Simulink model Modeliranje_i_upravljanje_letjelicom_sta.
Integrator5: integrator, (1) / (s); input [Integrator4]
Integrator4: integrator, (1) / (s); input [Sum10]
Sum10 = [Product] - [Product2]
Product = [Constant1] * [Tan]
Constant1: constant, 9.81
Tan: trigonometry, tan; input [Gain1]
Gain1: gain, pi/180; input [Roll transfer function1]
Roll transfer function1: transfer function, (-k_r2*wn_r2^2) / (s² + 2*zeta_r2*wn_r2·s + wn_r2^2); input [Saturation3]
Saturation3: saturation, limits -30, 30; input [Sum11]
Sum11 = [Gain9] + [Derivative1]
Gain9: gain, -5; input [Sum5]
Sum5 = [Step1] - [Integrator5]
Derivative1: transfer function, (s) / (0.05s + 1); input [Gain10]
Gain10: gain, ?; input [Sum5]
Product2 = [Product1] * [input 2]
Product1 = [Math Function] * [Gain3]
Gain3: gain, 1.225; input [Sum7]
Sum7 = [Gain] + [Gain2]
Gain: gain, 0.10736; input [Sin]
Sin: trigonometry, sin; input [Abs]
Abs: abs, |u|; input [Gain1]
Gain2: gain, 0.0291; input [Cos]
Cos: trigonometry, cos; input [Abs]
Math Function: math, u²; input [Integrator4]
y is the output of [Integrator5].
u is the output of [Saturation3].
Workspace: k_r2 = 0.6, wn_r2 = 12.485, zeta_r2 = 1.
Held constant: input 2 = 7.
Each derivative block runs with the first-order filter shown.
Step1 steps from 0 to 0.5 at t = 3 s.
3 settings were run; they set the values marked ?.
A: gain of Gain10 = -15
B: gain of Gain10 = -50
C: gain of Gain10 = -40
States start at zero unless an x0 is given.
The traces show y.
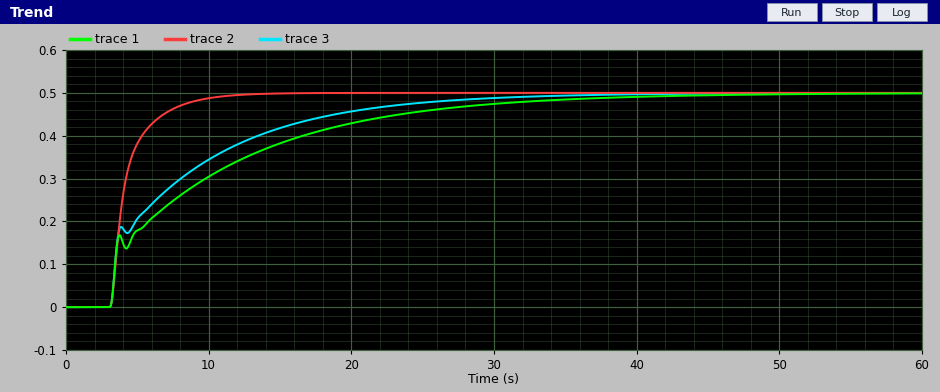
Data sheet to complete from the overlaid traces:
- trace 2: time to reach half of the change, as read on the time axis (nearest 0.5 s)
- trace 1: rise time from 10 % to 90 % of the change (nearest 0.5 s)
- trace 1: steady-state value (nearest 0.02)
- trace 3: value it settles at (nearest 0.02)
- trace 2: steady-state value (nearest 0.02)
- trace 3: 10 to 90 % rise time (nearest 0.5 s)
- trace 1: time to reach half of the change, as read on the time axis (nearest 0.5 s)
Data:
4.0 s
20.0 s
0.50
0.50
0.50
15.5 s
7.5 s
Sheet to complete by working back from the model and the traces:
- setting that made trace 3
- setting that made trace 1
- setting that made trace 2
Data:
C
B
A
